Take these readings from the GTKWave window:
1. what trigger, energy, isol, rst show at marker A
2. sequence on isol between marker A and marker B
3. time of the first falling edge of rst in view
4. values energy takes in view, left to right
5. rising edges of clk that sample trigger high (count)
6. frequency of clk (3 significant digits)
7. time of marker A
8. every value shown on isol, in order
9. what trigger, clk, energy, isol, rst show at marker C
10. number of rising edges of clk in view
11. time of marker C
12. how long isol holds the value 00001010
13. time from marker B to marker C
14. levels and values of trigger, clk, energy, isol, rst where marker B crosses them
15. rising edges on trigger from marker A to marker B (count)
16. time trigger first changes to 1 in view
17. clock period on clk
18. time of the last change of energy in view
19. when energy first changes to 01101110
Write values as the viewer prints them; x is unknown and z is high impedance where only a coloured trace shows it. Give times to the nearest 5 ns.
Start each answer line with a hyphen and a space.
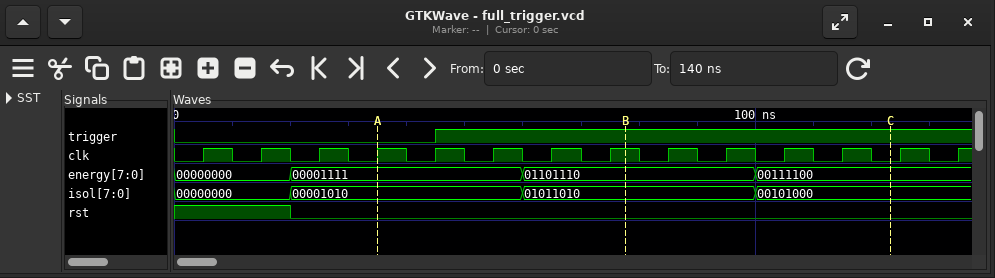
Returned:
- trigger=0, energy=00001111, isol=00001010, rst=0
- 00001010, 01011010
- 20 ns
- 00000000, 00001111, 01101110, 00111100
- 9
- 100 MHz
- 35 ns
- 00000000, 00001010, 01011010, 00101000
- trigger=1, clk=0, energy=00111100, isol=00101000, rst=0
- 14
- 125 ns
- 40 ns
- 45 ns
- trigger=1, clk=1, energy=01101110, isol=01011010, rst=0
- 1
- 45 ns
- 10 ns
- 100 ns
- 60 ns
